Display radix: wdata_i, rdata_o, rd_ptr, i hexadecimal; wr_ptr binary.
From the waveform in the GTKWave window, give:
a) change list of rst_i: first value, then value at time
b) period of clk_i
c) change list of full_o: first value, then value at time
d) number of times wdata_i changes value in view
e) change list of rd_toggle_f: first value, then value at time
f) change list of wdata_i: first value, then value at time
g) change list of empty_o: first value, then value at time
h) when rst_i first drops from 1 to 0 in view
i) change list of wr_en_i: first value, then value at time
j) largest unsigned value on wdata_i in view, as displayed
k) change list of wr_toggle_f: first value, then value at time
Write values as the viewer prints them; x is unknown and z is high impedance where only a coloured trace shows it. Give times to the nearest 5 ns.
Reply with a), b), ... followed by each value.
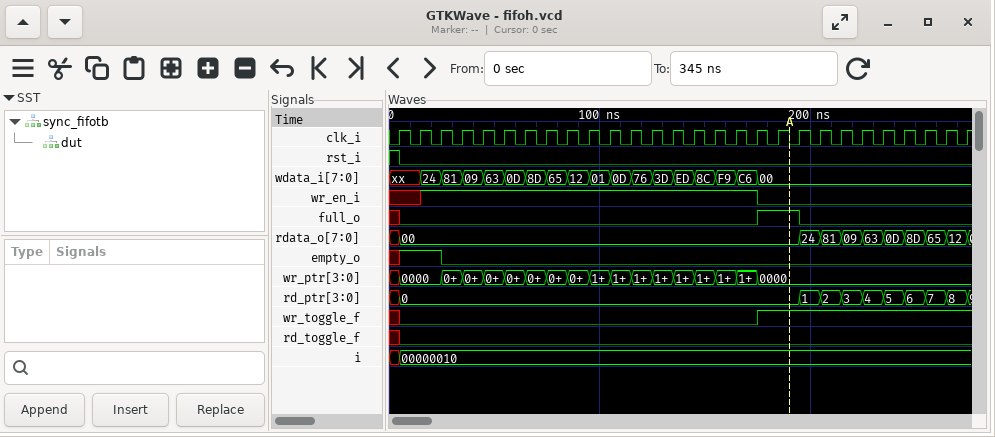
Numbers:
a) 1, 0 at 5 ns
b) 10 ns
c) x, 0 at 5 ns, 1 at 175 ns, 0 at 195 ns
d) 17
e) x, 0 at 5 ns
f) xx, 24 at 15 ns, 81 at 25 ns, 09 at 35 ns, 63 at 45 ns, 0D at 55 ns, 8D at 65 ns, 65 at 75 ns, 12 at 85 ns, 01 at 95 ns, 0D at 105 ns, 76 at 115 ns, 3D at 125 ns, ED at 135 ns, 8C at 145 ns, F9 at 155 ns, C6 at 165 ns, 00 at 175 ns
g) x, 1 at 5 ns, 0 at 25 ns
h) 5 ns
i) x, 1 at 15 ns, 0 at 175 ns
j) F9
k) x, 0 at 5 ns, 1 at 175 ns
